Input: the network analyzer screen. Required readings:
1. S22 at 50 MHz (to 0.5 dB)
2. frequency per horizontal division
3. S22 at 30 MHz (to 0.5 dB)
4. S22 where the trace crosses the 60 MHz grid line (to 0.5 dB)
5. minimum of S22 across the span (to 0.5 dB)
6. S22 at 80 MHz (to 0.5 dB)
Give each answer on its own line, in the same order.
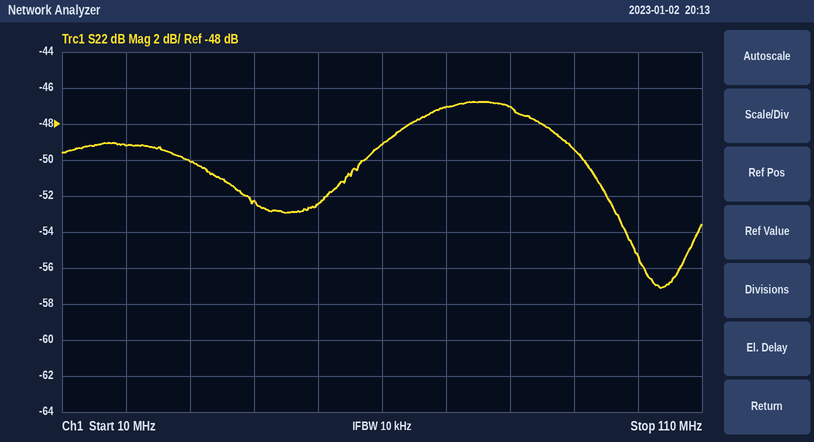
-52.5 dB
10 MHz
-50.0 dB
-49.0 dB
-57.0 dB
-47.0 dB
